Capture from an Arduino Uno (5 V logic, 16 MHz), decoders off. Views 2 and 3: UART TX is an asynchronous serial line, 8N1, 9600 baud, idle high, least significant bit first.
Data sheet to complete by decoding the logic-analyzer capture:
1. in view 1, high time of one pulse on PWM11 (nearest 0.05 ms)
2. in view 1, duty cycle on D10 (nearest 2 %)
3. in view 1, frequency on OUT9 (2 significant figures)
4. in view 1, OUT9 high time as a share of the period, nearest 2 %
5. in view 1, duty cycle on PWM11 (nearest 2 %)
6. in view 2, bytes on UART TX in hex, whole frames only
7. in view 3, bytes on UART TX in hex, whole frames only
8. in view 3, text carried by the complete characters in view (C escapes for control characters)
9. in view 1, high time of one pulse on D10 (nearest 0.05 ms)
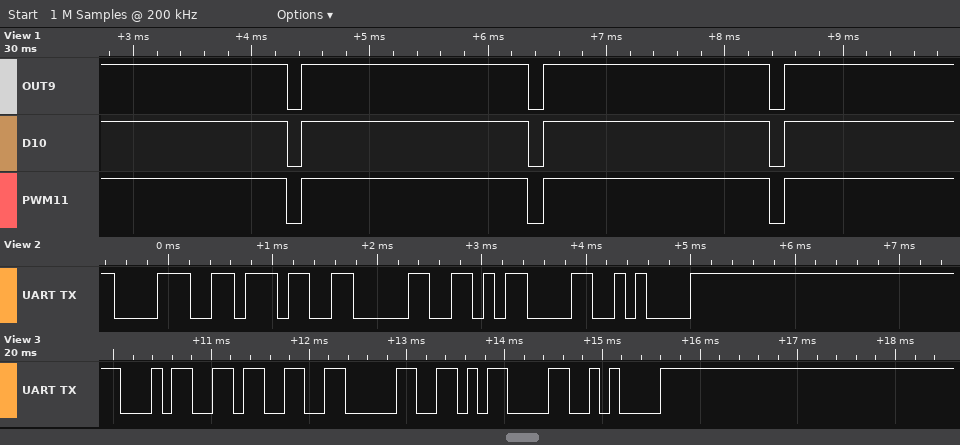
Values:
1.90 ms
94 %
490 Hz
94 %
94 %
38 37 30 0D 0A
34 33 30 0D 0A
"430\r\n"
1.90 ms
